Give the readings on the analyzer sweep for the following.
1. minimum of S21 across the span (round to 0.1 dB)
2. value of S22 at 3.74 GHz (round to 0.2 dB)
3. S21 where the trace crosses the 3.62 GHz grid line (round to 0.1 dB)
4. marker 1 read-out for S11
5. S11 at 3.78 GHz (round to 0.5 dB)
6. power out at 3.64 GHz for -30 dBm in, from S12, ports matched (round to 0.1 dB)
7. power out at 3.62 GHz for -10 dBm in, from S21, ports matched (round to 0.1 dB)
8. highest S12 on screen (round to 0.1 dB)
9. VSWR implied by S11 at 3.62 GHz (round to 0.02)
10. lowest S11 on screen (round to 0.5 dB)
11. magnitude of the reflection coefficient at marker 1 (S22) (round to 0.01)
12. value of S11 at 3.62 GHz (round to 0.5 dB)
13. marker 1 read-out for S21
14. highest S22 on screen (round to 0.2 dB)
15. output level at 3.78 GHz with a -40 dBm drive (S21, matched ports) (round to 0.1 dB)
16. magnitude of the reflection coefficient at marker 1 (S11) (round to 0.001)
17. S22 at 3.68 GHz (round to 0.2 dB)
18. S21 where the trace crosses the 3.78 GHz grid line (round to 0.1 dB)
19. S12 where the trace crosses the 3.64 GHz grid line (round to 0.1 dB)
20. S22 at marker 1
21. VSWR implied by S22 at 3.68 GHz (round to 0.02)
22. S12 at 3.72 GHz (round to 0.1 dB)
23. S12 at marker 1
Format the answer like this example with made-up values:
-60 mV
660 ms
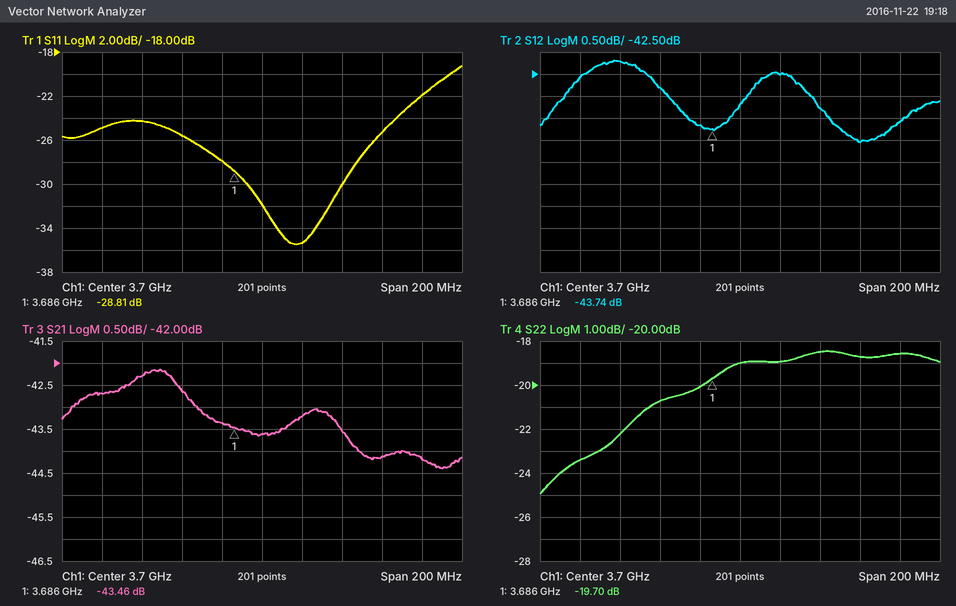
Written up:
-44.4 dB
-18.4 dB
-42.7 dB
-28.81 dB
-22.0 dB
-72.2 dBm
-52.7 dBm
-42.2 dB
1.12
-35.5 dB
0.10
-25.0 dB
-43.46 dB
-18.4 dB
-84.2 dBm
0.036
-20.0 dB
-44.2 dB
-42.2 dB
-19.70 dB
1.22
-42.5 dB
-43.74 dB
